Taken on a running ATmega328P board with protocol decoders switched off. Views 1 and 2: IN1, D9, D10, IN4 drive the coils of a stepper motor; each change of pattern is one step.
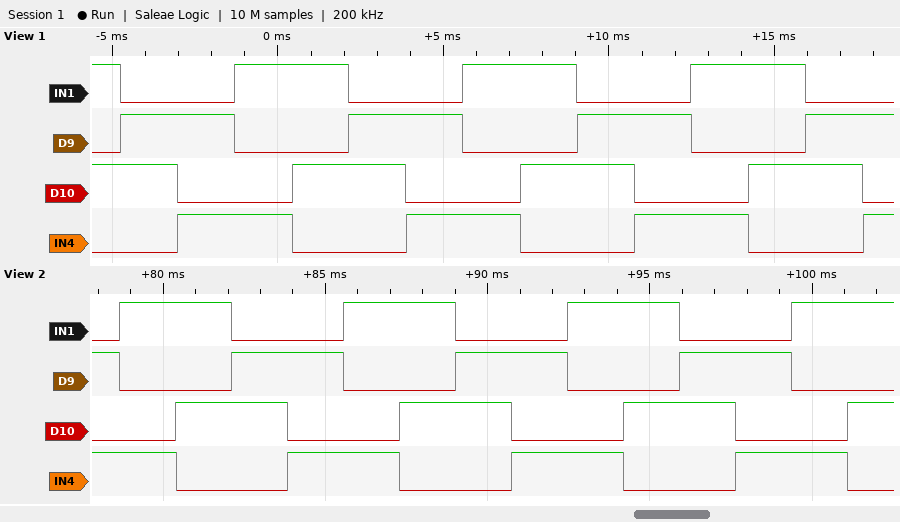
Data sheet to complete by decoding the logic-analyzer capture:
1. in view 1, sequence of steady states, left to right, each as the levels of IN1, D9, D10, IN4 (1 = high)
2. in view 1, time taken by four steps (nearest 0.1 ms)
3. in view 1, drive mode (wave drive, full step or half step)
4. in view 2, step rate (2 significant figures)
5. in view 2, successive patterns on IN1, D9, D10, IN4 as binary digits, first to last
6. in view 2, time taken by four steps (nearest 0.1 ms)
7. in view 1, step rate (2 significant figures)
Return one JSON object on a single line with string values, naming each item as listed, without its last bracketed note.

{"in view 1, sequence of steady states, left to right, each as the levels of IN1, D9, D10, IN4": "1010 0110 0101 1001 1010 0110 0101 1001 1010 0110 0101 1001 1010 0110 0101", "in view 1, time taken by four steps": "6.9 ms", "in view 1, drive mode": "full step", "in view 2, step rate": "580 steps/s", "in view 2, successive patterns on IN1, D9, D10, IN4 as binary digits, first to last": "0101 1001 1010 0110 0101 1001 1010 0110 0101 1001 1010 0110 0101 1001 1010", "in view 2, time taken by four steps": "6.9 ms", "in view 1, step rate": "580 steps/s"}
